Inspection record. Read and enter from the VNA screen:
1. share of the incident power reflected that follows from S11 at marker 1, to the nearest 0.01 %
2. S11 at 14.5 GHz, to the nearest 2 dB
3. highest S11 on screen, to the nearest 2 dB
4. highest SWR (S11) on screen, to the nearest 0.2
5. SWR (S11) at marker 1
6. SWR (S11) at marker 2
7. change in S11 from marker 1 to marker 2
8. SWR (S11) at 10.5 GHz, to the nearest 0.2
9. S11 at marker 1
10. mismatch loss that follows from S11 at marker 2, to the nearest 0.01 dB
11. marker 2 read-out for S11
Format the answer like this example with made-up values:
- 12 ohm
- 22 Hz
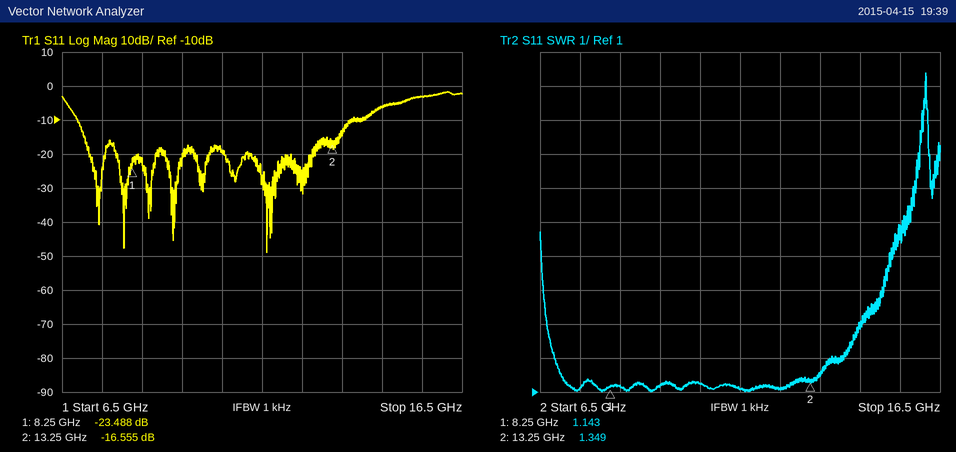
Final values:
- 0.45 %
- -6 dB
- -2 dB
- 10.4
- 1.143
- 1.349
- 6.933 dB
- 1.2
- -23.488 dB
- 0.10 dB
- -16.555 dB
